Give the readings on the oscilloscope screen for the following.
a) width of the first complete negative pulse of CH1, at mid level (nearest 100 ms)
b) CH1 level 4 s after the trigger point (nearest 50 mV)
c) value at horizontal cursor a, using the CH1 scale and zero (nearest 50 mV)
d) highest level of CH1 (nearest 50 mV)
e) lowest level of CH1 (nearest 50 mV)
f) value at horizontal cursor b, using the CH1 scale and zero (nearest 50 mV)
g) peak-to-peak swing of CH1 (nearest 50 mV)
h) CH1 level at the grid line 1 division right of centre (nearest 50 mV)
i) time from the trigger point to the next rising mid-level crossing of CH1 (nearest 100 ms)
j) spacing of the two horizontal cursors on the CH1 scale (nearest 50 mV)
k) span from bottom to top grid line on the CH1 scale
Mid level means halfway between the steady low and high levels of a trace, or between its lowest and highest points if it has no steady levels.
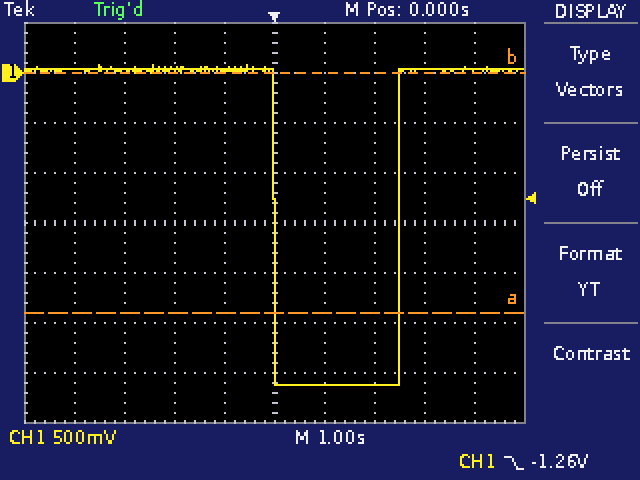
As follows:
2.5 s
50 mV
-2.40 V
100 mV
-3.10 V
0 mV
3.20 V
-3.10 V
2.5 s
2.40 V
4 V
